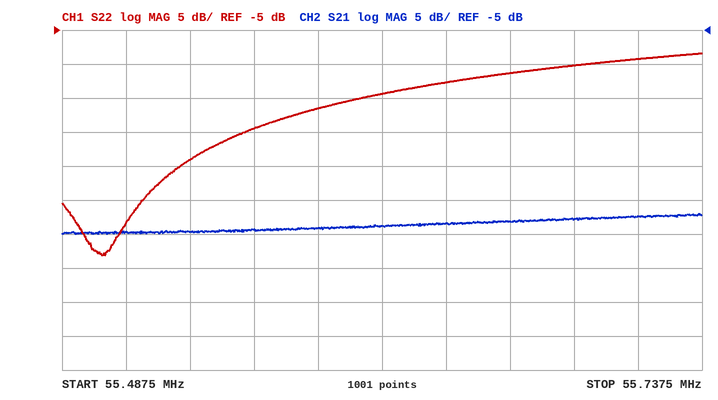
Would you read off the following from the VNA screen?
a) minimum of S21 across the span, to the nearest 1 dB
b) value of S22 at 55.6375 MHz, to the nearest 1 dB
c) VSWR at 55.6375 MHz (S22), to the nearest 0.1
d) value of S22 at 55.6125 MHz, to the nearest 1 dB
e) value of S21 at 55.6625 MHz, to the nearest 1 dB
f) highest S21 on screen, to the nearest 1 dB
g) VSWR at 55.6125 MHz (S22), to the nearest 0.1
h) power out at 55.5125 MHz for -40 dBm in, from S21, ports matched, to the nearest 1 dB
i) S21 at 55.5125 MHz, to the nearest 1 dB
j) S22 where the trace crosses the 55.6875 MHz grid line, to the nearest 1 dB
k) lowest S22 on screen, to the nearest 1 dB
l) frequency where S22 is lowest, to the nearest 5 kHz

-35 dB
-13 dB
1.6
-14 dB
-33 dB
-32 dB
1.5
-75 dBm
-35 dB
-10 dB
-38 dB
55.505 MHz
